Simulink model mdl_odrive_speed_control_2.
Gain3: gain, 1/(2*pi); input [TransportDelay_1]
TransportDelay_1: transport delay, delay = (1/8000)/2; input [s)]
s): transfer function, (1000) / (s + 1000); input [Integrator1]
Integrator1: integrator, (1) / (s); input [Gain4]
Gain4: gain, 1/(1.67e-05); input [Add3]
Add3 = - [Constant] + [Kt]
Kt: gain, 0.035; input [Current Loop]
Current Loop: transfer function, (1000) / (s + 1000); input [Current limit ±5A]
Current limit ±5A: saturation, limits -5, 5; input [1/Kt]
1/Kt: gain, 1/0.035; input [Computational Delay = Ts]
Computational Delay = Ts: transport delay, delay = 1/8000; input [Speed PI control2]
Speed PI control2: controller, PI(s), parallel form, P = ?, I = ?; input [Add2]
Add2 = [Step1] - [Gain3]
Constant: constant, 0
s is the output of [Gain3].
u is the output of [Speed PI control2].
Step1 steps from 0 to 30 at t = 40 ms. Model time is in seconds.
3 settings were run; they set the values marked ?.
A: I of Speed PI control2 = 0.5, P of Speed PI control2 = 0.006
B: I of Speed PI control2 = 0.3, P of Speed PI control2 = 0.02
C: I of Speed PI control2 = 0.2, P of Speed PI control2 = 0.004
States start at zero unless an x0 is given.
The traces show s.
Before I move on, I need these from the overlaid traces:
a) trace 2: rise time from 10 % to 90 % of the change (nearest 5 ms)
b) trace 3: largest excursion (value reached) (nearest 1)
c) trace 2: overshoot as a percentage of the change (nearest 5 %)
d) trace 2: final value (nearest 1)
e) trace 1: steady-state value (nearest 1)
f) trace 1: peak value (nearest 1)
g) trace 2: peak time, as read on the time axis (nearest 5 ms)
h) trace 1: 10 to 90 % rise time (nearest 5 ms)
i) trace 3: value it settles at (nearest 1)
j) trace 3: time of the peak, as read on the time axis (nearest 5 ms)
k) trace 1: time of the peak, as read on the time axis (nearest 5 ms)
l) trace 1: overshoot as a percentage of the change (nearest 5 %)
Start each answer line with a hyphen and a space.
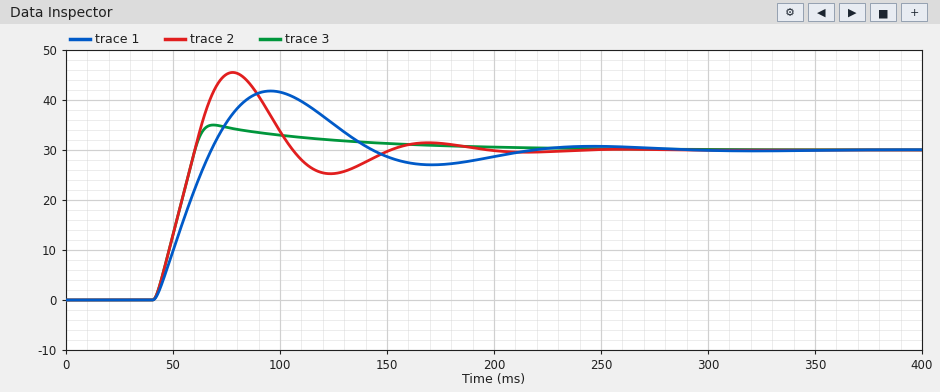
- 15 ms
- 35
- 50 %
- 30
- 30
- 42
- 80 ms
- 20 ms
- 30
- 70 ms
- 95 ms
- 40 %
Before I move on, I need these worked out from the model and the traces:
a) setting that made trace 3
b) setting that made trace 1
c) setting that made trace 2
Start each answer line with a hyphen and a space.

- B
- C
- A
